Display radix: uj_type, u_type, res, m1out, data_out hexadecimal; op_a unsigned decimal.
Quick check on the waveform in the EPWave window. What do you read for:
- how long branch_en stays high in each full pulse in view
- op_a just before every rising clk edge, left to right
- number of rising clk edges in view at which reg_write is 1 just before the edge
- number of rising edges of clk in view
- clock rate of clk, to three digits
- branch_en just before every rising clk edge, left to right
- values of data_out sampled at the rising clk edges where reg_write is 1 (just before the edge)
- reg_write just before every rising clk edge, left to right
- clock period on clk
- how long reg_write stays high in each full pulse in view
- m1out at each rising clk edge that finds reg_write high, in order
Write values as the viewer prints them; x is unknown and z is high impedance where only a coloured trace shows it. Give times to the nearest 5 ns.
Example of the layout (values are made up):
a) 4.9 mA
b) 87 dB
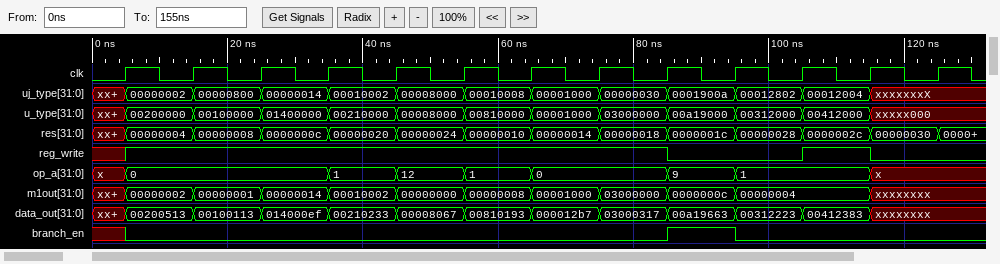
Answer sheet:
a) 10 ns
b) x, 0, 0, 0, 1, 12, 1, 0, 0, 9, 1, 1, x
c) 9
d) 13
e) 100 MHz
f) x 0 0 0 0 0 0 0 0 1 0 0 0
g) 00200513, 00100113, 014000ef, 00210233, 00008067, 00810193, 000012b7, 03000317, 00412383
h) x 1 1 1 1 1 1 1 1 0 0 1 0
i) 10 ns
j) 10 ns
k) 00000002, 00000001, 00000014, 00010002, 00000000, 00000008, 00001000, 03000000, 00000004
